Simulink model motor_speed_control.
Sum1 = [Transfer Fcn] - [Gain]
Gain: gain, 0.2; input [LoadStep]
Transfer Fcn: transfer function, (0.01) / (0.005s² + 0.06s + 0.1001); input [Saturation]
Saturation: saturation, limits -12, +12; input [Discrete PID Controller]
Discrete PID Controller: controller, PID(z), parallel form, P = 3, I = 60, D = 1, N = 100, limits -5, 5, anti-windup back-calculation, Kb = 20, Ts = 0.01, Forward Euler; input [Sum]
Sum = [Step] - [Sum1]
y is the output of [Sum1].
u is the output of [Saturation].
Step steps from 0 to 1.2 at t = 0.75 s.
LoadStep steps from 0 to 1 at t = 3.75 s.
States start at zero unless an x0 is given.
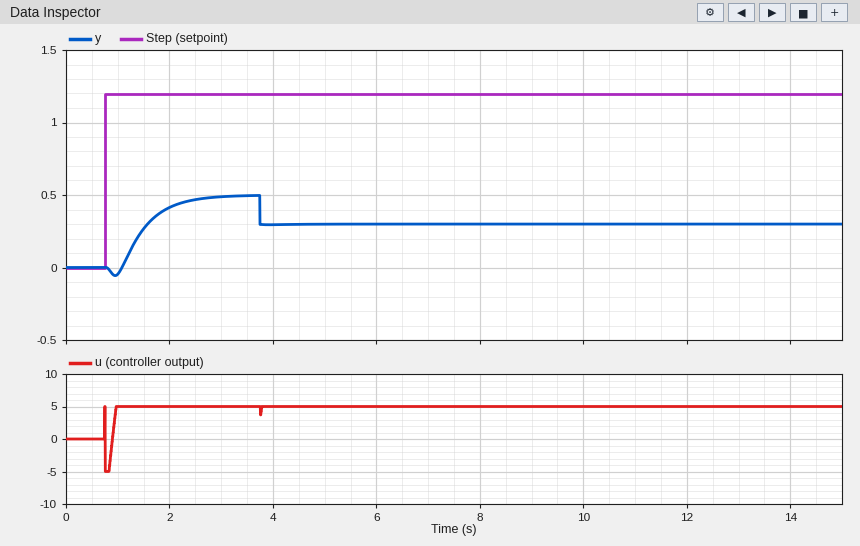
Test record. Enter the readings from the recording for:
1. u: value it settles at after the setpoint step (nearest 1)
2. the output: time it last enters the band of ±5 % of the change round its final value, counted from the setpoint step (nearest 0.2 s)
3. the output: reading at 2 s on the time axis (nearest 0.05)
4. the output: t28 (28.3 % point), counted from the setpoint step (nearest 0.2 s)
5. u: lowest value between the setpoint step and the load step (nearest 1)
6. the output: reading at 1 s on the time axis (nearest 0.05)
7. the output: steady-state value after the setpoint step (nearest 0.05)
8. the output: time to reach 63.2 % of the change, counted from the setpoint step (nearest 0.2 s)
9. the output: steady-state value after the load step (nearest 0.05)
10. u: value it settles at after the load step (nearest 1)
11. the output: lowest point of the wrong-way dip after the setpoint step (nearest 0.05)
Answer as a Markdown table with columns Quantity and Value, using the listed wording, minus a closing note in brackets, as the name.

| Quantity | Value |
|---|---|
| u: value it settles at after the setpoint step | 5 |
| the output: time it last enters the band of ±5 % of the change round its final value, counted from the setpoint step | 1.8 s |
| the output: reading at 2 s on the time axis | 0.40 |
| the output: t28 (28.3 % point), counted from the setpoint step | 0.6 s |
| u: lowest value between the setpoint step and the load step | -5 |
| the output: reading at 1 s on the time axis | -0.05 |
| the output: steady-state value after the setpoint step | 0.50 |
| the output: time to reach 63.2 % of the change, counted from the setpoint step | 0.8 s |
| the output: steady-state value after the load step | 0.30 |
| u: value it settles at after the load step | 5 |
| the output: lowest point of the wrong-way dip after the setpoint step | -0.05 |
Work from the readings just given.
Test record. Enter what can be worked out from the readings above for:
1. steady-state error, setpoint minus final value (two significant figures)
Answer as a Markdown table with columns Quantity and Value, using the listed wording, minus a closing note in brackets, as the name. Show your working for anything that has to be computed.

| Quantity | Value |
|---|---|
| steady-state error, setpoint minus final value | 1.2 - 0.5 = 0.70 |
